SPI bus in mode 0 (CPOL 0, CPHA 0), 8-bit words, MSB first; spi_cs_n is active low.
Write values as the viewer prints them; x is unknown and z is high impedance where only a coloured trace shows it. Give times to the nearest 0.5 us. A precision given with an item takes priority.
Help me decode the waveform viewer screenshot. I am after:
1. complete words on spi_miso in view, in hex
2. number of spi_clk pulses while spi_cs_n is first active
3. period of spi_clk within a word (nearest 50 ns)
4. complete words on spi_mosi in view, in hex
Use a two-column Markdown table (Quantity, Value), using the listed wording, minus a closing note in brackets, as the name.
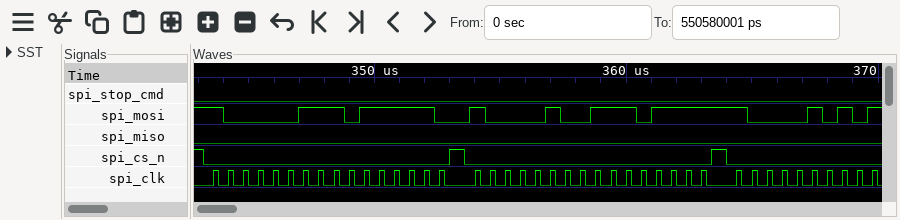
| Quantity | Value |
|---|---|
| complete words on spi_miso in view, in hex | 00, 00, 00, 00, 00 |
| number of spi_clk pulses while spi_cs_n is first active | 16 |
| period of spi_clk within a word | 600 ns |
| complete words on spi_mosi in view, in hex | 83, BE, 84, EF, 85 |
